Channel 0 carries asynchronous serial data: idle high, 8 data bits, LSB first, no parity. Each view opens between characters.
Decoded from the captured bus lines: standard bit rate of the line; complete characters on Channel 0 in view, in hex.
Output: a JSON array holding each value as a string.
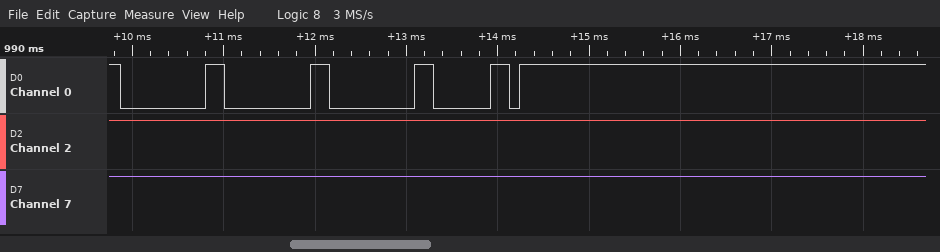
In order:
["9600 baud", "00, 00, 00, 60"]
